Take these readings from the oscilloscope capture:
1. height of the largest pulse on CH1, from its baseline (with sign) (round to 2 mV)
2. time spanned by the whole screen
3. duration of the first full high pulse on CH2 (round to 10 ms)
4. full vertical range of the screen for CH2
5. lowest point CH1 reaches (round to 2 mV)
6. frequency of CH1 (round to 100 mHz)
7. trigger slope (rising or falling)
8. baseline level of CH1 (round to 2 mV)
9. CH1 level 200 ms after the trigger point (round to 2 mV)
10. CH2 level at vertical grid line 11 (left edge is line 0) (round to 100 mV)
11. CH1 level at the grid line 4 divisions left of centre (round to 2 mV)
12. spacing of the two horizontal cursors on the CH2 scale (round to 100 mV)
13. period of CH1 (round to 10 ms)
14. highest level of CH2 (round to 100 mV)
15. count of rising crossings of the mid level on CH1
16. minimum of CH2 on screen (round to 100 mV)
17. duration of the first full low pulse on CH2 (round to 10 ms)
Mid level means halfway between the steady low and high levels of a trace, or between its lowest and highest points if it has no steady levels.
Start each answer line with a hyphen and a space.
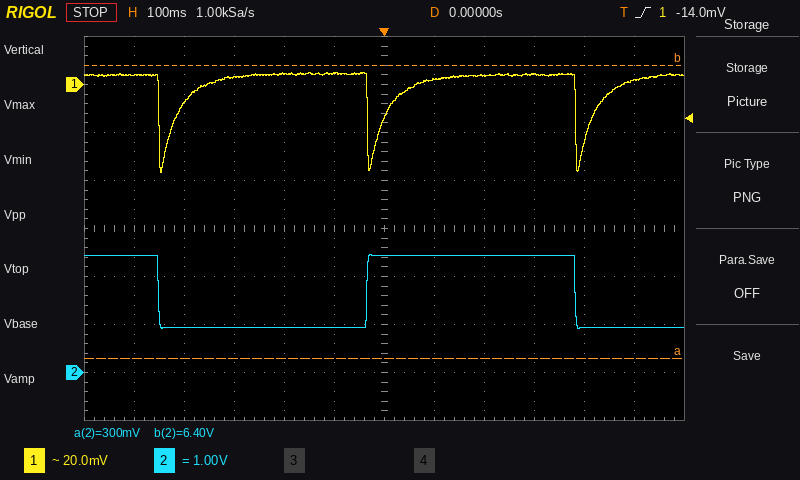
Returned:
- -40 mV
- 1.2 s
- 420 ms
- 8 V
- -36 mV
- 2.4 Hz
- rising
- 4 mV
- 4 mV
- 900 mV
- -8 mV
- 6.1 V
- 420 ms
- 2.5 V
- 3
- 900 mV
- 420 ms
